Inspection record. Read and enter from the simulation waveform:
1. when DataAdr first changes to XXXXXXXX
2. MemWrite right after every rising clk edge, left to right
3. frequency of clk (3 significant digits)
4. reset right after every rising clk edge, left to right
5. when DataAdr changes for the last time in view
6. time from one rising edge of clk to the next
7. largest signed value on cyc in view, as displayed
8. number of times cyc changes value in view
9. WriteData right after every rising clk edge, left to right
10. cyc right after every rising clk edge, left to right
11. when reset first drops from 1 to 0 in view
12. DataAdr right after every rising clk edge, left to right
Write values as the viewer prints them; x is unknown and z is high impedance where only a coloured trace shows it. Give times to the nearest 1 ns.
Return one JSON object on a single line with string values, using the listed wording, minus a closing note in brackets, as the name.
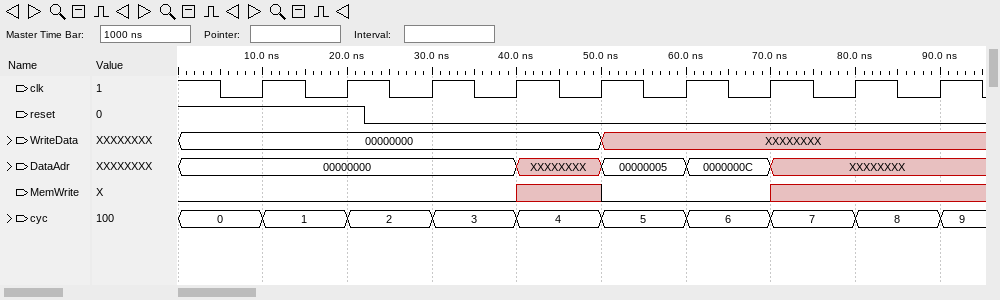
{"when DataAdr first changes to XXXXXXXX": "40 ns", "MemWrite right after every rising clk edge, left to right": "0 0 0 x 0 0 x x x", "frequency of clk": "100 MHz", "reset right after every rising clk edge, left to right": "1 1 0 0 0 0 0 0 0", "when DataAdr changes for the last time in view": "70 ns", "time from one rising edge of clk to the next": "10 ns", "largest signed value on cyc in view, as displayed": "9", "number of times cyc changes value in view": "9", "WriteData right after every rising clk edge, left to right": "00000000, 00000000, 00000000, 00000000, XXXXXXXX, XXXXXXXX, XXXXXXXX, XXXXXXXX, XXXXXXXX", "cyc right after every rising clk edge, left to right": "1, 2, 3, 4, 5, 6, 7, 8, 9", "when reset first drops from 1 to 0 in view": "22 ns", "DataAdr right after every rising clk edge, left to right": "00000000, 00000000, 00000000, XXXXXXXX, 00000005, 0000000C, XXXXXXXX, XXXXXXXX, XXXXXXXX"}
